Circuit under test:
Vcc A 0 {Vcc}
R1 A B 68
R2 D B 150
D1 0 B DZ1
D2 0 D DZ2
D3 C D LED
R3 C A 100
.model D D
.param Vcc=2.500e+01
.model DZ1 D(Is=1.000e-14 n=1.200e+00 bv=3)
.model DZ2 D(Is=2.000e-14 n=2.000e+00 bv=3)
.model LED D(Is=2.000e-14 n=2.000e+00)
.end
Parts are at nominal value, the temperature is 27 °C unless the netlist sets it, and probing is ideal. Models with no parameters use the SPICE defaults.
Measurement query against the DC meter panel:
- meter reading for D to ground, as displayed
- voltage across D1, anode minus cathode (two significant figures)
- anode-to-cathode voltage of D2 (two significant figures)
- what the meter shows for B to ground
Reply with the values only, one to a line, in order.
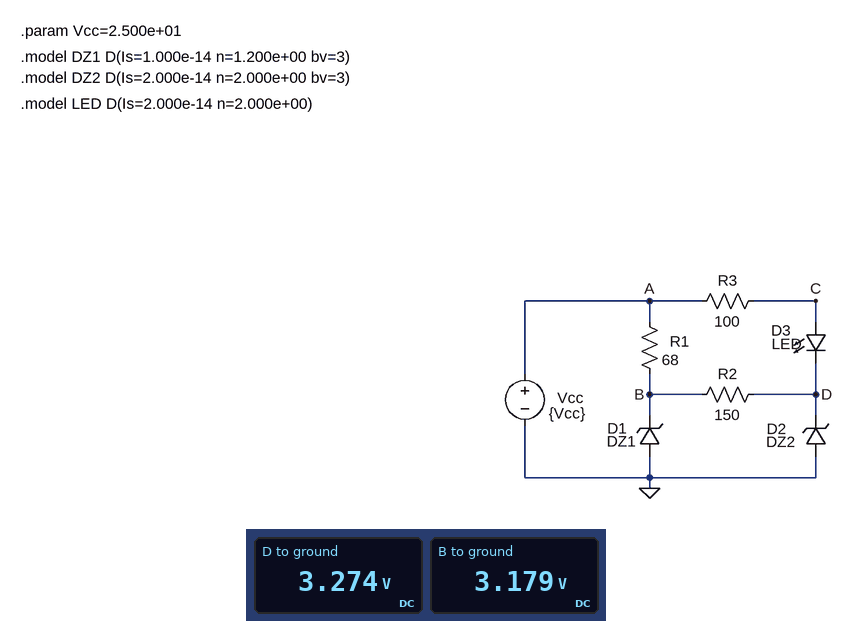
3.274 V
-3.2 V
-3.3 V
3.179 V
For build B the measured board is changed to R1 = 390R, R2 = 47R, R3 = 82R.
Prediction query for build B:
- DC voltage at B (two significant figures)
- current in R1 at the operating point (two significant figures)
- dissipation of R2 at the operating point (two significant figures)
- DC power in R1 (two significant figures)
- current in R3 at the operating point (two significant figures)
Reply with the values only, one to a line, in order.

3.1 V
56 mA
530 µW
1.2 W
250 mA
